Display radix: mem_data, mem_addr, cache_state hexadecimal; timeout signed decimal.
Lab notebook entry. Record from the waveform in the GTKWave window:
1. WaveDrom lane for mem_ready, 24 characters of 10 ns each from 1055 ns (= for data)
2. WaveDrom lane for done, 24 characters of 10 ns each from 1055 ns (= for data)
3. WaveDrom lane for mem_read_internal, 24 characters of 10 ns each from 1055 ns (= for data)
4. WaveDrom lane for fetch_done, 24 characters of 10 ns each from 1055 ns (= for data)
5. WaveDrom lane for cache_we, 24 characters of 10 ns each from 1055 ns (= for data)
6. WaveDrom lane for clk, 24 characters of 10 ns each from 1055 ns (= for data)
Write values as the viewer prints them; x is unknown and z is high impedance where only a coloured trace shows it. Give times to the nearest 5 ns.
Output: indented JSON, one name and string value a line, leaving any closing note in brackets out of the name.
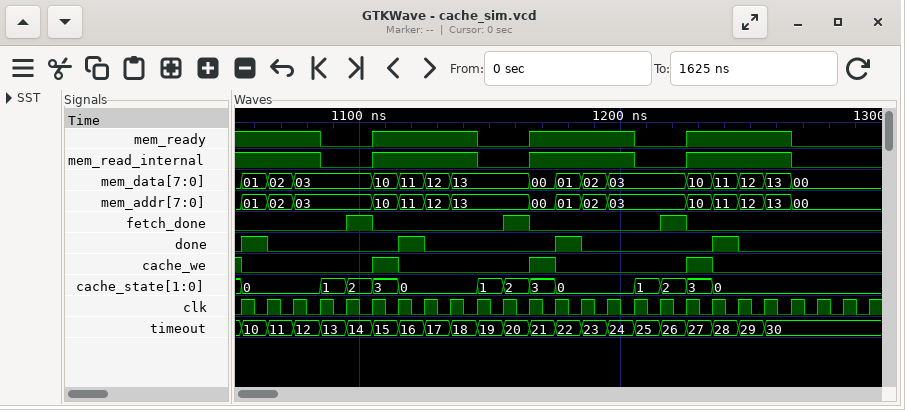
{
  "WaveDrom lane for mem_ready, 24 characters of 10 ns each from 1055 ns": "{name: 'mem_ready', wave: '1..0.1...0.1...0.1...0..'}",
  "WaveDrom lane for done, 24 characters of 10 ns each from 1055 ns": "{name: 'done', wave: '10....10....10....10....'}",
  "WaveDrom lane for mem_read_internal, 24 characters of 10 ns each from 1055 ns": "{name: 'mem_read_internal', wave: '1..0.1...0.1...0.1...0..'}",
  "WaveDrom lane for fetch_done, 24 characters of 10 ns each from 1055 ns": "{name: 'fetch_done', wave: '0...10....10....10......'}",
  "WaveDrom lane for cache_we, 24 characters of 10 ns each from 1055 ns": "{name: 'cache_we', wave: '0....10....10....10.....'}",
  "WaveDrom lane for clk, 24 characters of 10 ns each from 1055 ns": "{name: 'clk', wave: 'p.......................'}"
}
